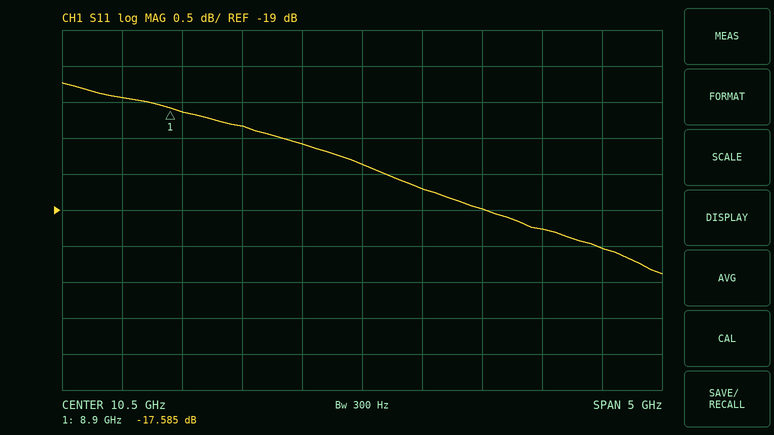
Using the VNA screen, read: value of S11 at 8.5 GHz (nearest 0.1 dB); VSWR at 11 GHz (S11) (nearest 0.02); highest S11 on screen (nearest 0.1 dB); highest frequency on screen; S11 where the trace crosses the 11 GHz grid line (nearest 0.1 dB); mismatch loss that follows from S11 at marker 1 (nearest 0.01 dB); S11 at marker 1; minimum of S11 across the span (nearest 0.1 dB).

-17.4 dB
1.26
-17.2 dB
13 GHz
-18.7 dB
0.08 dB
-17.585 dB
-19.9 dB
